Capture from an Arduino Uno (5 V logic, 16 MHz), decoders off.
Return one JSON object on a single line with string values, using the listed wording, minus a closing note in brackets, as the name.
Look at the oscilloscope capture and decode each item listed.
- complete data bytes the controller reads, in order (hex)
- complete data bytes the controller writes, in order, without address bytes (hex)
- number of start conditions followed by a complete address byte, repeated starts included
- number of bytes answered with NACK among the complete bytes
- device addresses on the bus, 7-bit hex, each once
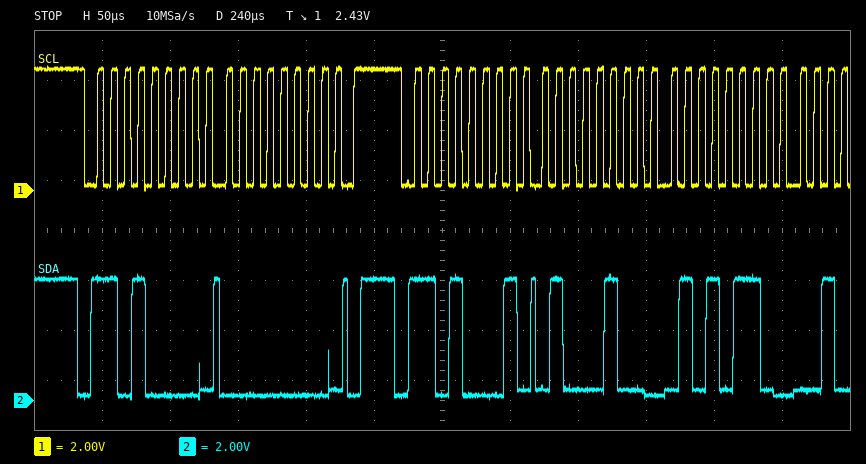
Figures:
{"complete data bytes the controller reads, in order": "44 56", "complete data bytes the controller writes, in order, without address bytes": "00", "number of start conditions followed by a complete address byte, repeated starts included": "2", "number of bytes answered with NACK among the complete bytes": "0", "device addresses on the bus, 7-bit hex, each once": "0x68"}
